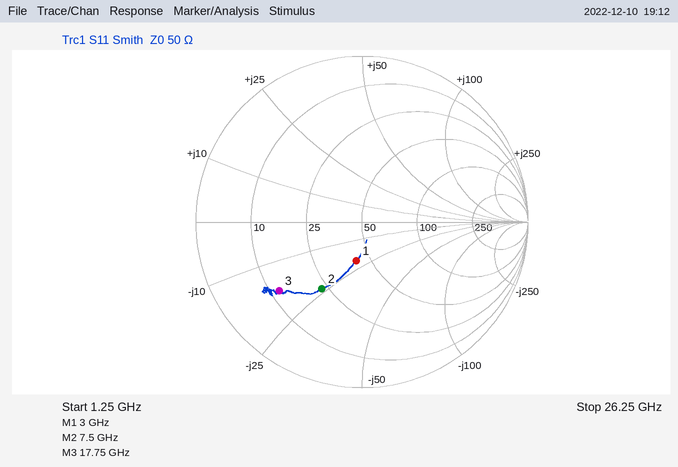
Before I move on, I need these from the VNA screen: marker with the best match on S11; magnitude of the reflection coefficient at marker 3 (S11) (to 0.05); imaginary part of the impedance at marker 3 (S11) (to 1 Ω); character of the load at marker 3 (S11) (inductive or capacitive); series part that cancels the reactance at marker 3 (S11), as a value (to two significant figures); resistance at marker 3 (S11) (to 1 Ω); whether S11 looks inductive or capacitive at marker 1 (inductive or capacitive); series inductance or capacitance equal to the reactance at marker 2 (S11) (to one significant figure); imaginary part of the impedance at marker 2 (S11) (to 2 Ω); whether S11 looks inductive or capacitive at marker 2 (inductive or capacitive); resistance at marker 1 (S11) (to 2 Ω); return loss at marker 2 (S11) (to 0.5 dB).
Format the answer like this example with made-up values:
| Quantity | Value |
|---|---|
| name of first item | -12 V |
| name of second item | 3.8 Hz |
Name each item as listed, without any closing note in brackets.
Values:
| Quantity | Value |
|---|---|
| marker with the best match on S11 | marker 1 |
| magnitude of the reflection coefficient at marker 3 (S11) | 0.65 |
| imaginary part of the impedance at marker 3 (S11) | -17 Ω |
| character of the load at marker 3 (S11) | capacitive |
| series part that cancels the reactance at marker 3 (S11), as a value | 150 pH |
| resistance at marker 3 (S11) | 12 Ω |
| whether S11 looks inductive or capacitive at marker 1 | capacitive |
| series inductance or capacitance equal to the reactance at marker 2 (S11) | 900 fF |
| imaginary part of the impedance at marker 2 (S11) | -24 Ω |
| whether S11 looks inductive or capacitive at marker 2 | capacitive |
| resistance at marker 1 (S11) | 42 Ω |
| return loss at marker 2 (S11) | 6.5 dB |
